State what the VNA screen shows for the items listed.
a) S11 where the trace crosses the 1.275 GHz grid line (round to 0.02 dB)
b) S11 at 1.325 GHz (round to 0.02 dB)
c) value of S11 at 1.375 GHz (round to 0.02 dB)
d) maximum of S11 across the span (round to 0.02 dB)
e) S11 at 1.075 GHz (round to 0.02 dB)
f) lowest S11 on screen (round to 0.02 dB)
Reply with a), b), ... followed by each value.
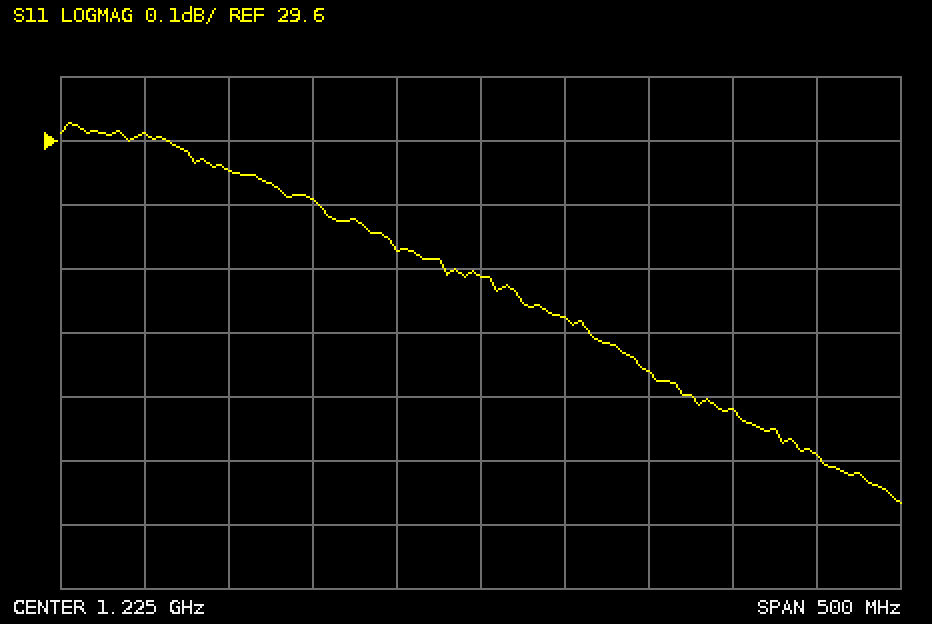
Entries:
a) 29.32 dB
b) 29.24 dB
c) 29.18 dB
d) 29.62 dB
e) 29.56 dB
f) 29.04 dB
